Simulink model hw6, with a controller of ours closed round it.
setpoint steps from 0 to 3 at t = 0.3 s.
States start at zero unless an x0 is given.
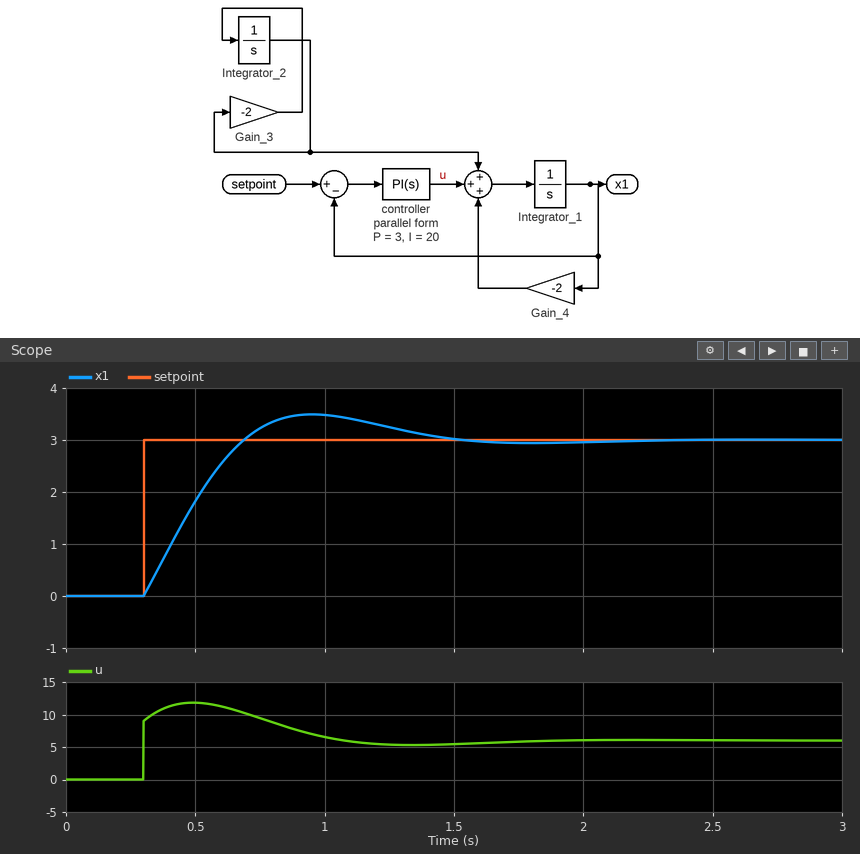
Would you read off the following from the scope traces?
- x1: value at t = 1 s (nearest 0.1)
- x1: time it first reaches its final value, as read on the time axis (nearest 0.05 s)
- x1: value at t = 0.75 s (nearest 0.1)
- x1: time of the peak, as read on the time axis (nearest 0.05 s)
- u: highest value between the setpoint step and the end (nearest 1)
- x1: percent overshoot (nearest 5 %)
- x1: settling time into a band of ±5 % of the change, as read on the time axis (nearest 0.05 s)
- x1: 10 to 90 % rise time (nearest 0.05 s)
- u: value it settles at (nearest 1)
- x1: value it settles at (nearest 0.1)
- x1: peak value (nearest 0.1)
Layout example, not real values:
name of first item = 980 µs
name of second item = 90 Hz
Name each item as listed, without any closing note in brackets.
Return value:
x1: value at t = 1 s = 3.5
x1: time it first reaches its final value, as read on the time axis = 0.70 s
x1: value at t = 0.75 s = 3.2
x1: time of the peak, as read on the time axis = 0.95 s
u: highest value between the setpoint step and the end = 12
x1: percent overshoot = 15 %
x1: settling time into a band of ±5 % of the change, as read on the time axis = 1.35 s
x1: 10 to 90 % rise time = 0.30 s
u: value it settles at = 6
x1: value it settles at = 3.0
x1: peak value = 3.5
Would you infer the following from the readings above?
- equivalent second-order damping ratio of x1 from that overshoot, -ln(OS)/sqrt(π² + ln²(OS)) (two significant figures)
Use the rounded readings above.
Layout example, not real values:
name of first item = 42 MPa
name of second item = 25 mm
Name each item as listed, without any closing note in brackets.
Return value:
equivalent second-order damping ratio of x1 from that overshoot, -ln(OS)/sqrt(π² + ln²(OS)) = 0.52
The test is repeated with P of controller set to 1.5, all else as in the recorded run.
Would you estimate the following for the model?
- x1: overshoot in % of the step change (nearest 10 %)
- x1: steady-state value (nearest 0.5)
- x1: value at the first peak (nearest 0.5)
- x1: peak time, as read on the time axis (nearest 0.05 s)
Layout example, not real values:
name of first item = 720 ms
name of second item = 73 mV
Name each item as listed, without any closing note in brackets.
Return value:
x1: overshoot in % of the step change = 30 %
x1: steady-state value = 3.0
x1: value at the first peak = 4.0
x1: peak time, as read on the time axis = 1.00 s
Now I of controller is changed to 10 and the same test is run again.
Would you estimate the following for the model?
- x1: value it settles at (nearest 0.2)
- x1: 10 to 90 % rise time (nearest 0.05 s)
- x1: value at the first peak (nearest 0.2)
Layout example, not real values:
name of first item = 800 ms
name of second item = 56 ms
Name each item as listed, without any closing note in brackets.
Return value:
x1: value it settles at = 3.0
x1: 10 to 90 % rise time = 0.45 s
x1: value at the first peak = 3.2
